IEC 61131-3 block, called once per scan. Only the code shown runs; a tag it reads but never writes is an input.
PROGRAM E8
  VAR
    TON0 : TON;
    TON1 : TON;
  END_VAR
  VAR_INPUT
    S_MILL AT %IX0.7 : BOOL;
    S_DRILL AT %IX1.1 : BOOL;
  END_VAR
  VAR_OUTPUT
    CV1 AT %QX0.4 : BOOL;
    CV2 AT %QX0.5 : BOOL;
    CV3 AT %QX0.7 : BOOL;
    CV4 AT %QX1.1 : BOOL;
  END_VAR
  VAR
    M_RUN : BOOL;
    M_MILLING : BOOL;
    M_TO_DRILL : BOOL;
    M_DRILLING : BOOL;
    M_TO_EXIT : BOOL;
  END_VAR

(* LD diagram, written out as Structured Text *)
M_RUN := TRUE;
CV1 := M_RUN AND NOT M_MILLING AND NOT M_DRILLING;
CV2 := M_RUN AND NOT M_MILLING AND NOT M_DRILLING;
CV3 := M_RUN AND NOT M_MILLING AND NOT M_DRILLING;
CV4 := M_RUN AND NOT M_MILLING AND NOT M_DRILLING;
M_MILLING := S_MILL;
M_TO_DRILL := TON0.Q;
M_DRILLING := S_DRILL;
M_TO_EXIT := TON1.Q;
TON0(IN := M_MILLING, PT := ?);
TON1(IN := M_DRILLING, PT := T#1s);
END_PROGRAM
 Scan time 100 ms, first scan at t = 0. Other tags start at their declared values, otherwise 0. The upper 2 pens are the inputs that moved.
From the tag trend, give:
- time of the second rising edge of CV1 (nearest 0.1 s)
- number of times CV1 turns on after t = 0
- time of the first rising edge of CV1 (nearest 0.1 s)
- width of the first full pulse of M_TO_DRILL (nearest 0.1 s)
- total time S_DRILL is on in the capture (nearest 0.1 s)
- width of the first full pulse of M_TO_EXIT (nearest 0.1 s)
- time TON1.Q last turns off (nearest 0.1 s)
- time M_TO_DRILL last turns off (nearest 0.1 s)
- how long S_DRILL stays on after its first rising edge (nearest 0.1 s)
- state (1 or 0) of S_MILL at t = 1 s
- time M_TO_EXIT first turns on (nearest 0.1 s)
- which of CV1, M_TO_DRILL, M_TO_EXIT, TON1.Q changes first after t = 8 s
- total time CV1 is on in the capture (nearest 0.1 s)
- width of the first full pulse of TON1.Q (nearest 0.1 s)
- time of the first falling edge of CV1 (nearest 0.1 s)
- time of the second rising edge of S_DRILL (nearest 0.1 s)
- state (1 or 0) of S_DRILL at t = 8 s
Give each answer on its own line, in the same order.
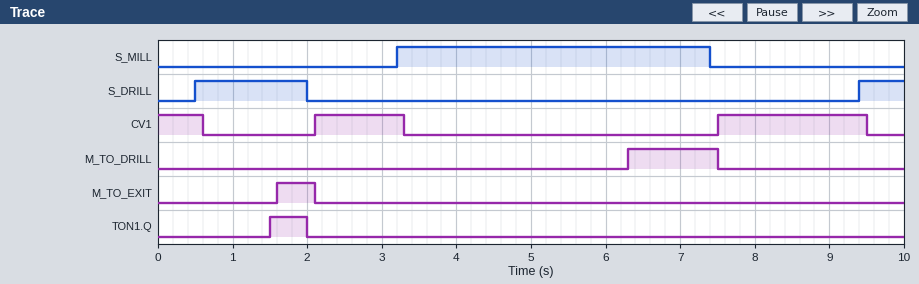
7.5 s
2
2.1 s
1.2 s
2.1 s
0.5 s
2.0 s
7.5 s
1.5 s
0
1.6 s
CV1
3.8 s
0.5 s
0.6 s
9.4 s
0
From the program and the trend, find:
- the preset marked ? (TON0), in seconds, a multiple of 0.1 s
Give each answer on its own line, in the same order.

3.0 s
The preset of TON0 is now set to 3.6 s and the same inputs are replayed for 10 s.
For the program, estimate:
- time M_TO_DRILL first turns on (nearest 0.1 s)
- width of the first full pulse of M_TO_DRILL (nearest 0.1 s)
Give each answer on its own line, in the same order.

6.9 s
0.6 s
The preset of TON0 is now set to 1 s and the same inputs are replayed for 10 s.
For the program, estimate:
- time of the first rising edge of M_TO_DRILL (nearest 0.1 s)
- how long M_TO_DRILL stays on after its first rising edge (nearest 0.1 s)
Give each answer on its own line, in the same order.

4.3 s
3.2 s
